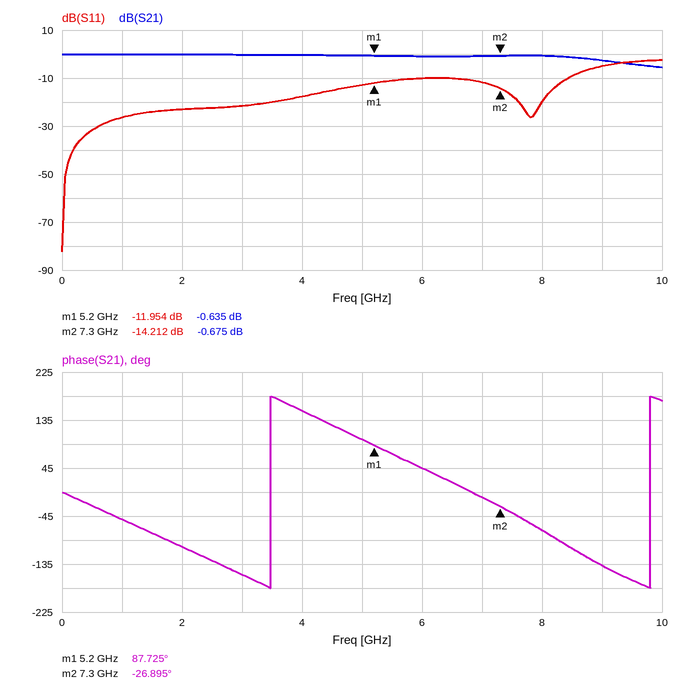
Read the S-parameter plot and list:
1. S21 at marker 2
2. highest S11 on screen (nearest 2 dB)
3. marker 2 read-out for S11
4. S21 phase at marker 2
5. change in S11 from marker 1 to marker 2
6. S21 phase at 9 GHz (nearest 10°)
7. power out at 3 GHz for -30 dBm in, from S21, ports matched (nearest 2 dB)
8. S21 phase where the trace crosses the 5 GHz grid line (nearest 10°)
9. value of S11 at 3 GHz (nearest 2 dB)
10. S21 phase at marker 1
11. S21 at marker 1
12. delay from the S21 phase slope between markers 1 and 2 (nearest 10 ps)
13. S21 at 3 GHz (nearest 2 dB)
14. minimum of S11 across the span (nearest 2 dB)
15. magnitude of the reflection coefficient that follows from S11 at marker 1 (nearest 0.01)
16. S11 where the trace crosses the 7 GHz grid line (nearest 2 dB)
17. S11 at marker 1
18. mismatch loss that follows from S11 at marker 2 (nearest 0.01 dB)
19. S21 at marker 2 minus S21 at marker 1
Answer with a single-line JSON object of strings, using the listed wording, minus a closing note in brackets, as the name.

{"S21 at marker 2": "-0.675 dB", "highest S11 on screen": "-2 dB", "marker 2 read-out for S11": "-14.212 dB", "S21 phase at marker 2": "-26.895°", "change in S11 from marker 1 to marker 2": "-2.258 dB", "S21 phase at 9 GHz": "-140°", "power out at 3 GHz for -30 dBm in, from S21, ports matched": "-30 dBm", "S21 phase where the trace crosses the 5 GHz grid line": "100°", "value of S11 at 3 GHz": "-22 dB", "S21 phase at marker 1": "87.725°", "S21 at marker 1": "-0.635 dB", "delay from the S21 phase slope between markers 1 and 2": "150 ps", "S21 at 3 GHz": "0 dB", "minimum of S11 across the span": "-82 dB", "magnitude of the reflection coefficient that follows from S11 at marker 1": "0.25", "S11 where the trace crosses the 7 GHz grid line": "-12 dB", "S11 at marker 1": "-11.954 dB", "mismatch loss that follows from S11 at marker 2": "0.17 dB", "S21 at marker 2 minus S21 at marker 1": "-0.040 dB"}
